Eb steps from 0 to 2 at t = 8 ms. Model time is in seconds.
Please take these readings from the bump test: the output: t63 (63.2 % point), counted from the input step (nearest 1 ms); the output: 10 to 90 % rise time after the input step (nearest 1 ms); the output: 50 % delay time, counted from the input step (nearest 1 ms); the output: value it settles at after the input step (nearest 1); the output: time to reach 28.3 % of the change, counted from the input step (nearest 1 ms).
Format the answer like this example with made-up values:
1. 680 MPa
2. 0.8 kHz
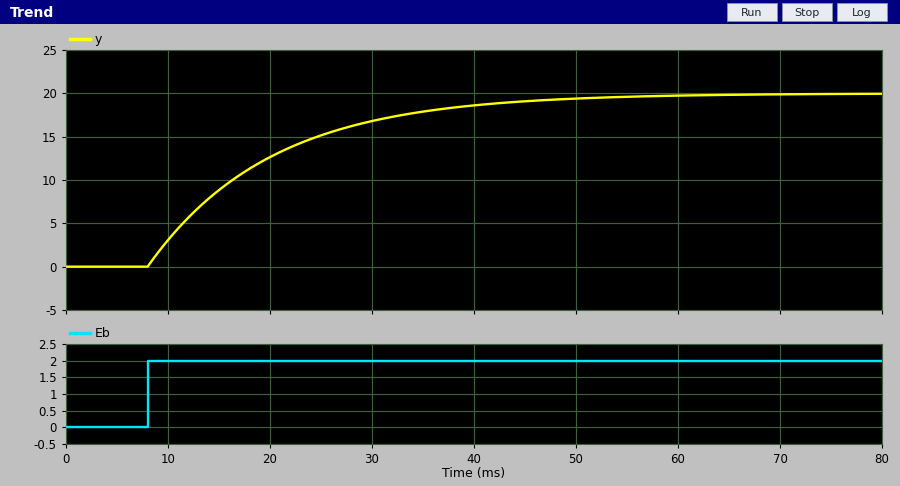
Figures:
1. 12 ms
2. 26 ms
3. 8 ms
4. 20
5. 4 ms
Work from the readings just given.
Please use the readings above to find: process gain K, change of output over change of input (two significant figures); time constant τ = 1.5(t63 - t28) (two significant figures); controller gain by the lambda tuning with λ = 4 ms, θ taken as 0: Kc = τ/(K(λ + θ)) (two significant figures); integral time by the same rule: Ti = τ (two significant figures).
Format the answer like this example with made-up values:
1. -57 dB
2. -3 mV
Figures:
1. 10
2. 12 ms
3. 0.30
4. 12 ms
